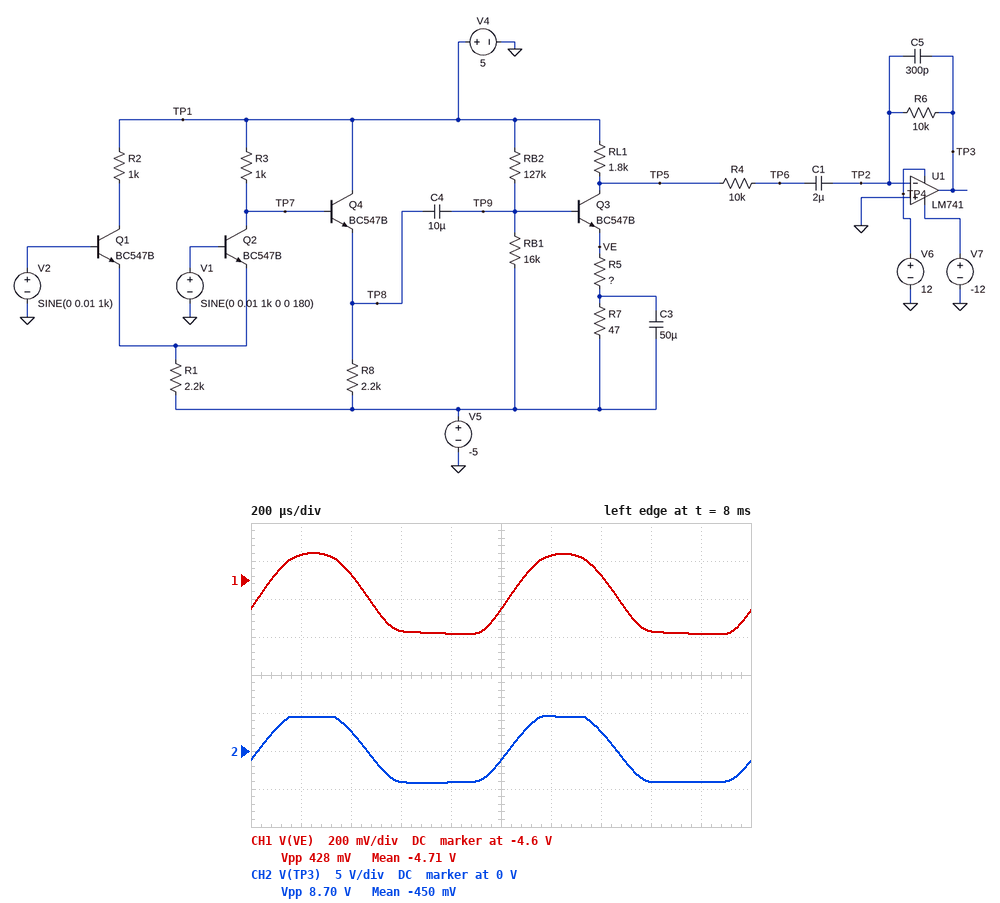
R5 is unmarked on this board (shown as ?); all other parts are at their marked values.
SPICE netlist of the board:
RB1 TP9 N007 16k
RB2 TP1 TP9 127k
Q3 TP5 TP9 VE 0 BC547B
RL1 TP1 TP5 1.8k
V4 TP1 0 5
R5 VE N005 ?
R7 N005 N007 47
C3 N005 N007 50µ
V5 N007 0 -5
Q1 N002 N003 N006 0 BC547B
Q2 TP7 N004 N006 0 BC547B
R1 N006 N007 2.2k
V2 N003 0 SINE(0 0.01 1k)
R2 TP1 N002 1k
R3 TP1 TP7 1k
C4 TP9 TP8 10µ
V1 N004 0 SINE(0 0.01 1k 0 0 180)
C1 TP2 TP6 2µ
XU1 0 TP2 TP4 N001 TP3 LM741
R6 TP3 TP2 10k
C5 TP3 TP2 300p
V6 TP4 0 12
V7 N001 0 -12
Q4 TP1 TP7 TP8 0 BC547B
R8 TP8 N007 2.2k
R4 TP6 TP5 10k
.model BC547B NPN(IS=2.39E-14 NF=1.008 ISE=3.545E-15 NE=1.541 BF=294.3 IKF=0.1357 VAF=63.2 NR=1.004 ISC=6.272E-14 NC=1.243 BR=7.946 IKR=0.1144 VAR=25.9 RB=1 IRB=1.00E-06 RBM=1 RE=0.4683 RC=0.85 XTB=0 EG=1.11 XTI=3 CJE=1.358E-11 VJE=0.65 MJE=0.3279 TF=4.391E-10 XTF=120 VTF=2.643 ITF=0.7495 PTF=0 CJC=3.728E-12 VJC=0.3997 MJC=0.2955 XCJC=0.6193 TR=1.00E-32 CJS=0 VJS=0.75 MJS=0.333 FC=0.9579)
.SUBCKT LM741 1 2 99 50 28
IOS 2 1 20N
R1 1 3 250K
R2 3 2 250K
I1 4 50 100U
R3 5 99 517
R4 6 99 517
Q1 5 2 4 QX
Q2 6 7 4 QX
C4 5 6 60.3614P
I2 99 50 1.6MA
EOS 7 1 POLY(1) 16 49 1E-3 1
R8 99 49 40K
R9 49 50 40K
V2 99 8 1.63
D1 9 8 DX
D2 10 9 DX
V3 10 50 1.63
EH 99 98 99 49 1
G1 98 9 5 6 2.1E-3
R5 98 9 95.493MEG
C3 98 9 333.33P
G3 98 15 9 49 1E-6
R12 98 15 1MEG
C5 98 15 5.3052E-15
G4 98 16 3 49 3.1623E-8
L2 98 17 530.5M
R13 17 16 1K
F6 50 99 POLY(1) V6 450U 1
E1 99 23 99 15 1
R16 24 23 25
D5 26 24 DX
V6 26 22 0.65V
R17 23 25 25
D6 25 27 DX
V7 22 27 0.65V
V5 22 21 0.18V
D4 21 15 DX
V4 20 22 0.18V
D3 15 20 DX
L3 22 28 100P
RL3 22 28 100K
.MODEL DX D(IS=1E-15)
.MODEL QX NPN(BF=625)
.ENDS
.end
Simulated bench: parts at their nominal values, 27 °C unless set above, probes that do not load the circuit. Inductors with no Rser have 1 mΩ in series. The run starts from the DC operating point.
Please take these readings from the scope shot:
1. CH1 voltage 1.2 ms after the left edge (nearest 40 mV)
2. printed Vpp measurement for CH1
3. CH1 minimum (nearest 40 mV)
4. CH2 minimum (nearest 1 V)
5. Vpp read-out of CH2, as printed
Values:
-4.48 V
428 mV
-4.88 V
-4 V
8.70 V
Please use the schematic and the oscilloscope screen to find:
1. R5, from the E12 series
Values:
68 Ω
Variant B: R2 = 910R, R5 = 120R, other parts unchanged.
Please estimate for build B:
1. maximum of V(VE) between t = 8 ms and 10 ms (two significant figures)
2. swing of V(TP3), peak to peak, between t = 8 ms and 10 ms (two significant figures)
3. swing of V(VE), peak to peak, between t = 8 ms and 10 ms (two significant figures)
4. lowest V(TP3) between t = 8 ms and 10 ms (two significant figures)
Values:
-4.3 V
7.2 V
570 mV
-3.3 V
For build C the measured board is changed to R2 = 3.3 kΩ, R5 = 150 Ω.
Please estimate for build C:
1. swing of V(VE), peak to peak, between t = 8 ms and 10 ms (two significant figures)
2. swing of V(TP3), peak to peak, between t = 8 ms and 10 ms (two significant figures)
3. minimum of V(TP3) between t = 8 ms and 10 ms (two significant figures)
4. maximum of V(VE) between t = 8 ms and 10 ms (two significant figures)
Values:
590 mV
5.9 V
-2.8 V
-4.3 V
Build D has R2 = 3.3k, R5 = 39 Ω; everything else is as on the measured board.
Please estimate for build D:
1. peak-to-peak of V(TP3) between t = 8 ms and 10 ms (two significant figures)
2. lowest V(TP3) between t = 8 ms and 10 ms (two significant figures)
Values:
8.9 V
-4.6 V
